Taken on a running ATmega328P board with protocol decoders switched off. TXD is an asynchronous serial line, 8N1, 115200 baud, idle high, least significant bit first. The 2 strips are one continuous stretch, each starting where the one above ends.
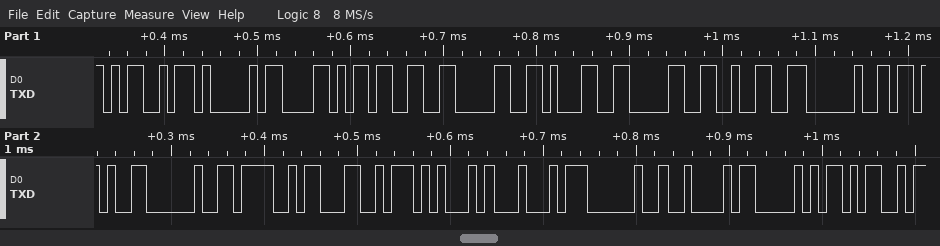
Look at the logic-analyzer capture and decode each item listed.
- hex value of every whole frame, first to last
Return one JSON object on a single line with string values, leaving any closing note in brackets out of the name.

{"hex value of every whole frame, first to last": "4D 41 58 33 30 31 30 32 20 2B 20 4F 4C 45 44 20 42 50 4D"}
